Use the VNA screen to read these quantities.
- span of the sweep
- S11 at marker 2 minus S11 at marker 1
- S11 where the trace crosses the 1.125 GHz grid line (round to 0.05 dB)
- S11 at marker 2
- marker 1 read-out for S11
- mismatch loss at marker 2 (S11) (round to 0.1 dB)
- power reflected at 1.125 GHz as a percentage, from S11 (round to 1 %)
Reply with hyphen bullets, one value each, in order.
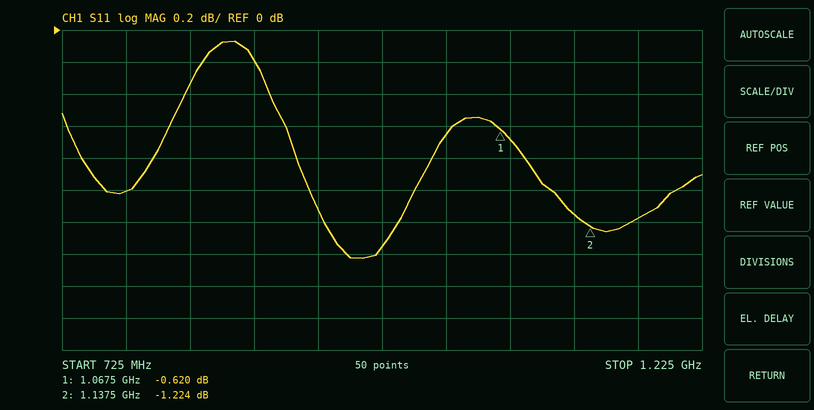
- 500 MHz
- -0.604 dB
- -1.15 dB
- -1.224 dB
- -0.620 dB
- 6.1 dB
- 77 %
